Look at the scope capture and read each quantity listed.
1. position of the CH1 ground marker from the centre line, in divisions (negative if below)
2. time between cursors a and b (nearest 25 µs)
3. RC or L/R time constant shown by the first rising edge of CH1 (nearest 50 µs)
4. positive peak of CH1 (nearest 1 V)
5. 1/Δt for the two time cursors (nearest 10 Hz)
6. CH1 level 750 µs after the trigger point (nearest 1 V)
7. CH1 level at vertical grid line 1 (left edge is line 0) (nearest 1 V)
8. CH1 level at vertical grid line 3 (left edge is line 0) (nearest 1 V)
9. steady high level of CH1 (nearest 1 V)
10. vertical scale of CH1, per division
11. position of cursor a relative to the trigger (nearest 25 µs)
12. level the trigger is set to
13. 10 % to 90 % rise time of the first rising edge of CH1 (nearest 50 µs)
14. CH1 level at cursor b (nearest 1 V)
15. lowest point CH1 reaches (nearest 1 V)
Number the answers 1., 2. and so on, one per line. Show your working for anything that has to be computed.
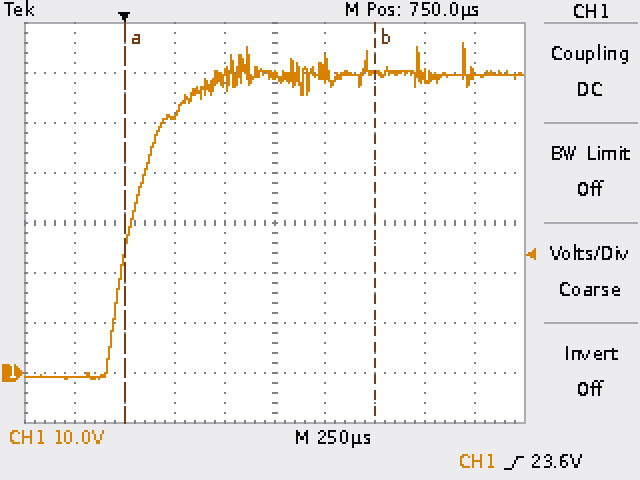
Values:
1. -3.0 div
2. 1.250 ms
3. 350 µs / 2.2 ≈ 159 µs, so 150 µs to the nearest 50 µs
4. 66 V
5. 1 / 1.250 ms ≈ 800 Hz
6. 60 V
7. -1 V
8. 52 V
9. 60 V
10. 10 V
11. 0 µs
12. 23.6 V
13. 350 µs
14. 60 V
15. -1 V
